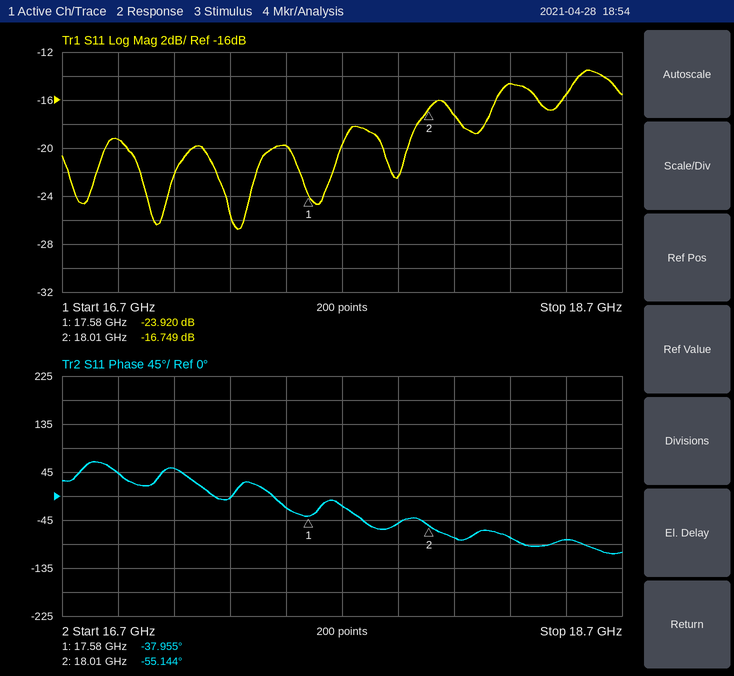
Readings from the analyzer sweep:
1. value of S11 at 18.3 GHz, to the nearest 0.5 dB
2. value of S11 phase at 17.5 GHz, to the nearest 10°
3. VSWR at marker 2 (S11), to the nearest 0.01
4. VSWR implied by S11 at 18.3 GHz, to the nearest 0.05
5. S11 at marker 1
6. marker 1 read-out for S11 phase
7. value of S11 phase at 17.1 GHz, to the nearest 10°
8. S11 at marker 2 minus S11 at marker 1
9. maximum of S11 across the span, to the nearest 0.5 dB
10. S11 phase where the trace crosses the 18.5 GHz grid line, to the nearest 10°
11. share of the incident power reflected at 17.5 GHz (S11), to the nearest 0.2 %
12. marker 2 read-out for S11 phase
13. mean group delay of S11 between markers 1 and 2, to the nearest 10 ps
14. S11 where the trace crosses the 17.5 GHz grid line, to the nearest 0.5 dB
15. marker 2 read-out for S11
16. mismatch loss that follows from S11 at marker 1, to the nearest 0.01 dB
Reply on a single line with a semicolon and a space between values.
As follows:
-14.5 dB; -20°; 1.34; 1.45; -23.920 dB; -37.955°; 50°; 7.171 dB; -13.5 dB; -80°; 1.0 %; -55.144°; 110 ps; -20.0 dB; -16.749 dB; 0.02 dB
